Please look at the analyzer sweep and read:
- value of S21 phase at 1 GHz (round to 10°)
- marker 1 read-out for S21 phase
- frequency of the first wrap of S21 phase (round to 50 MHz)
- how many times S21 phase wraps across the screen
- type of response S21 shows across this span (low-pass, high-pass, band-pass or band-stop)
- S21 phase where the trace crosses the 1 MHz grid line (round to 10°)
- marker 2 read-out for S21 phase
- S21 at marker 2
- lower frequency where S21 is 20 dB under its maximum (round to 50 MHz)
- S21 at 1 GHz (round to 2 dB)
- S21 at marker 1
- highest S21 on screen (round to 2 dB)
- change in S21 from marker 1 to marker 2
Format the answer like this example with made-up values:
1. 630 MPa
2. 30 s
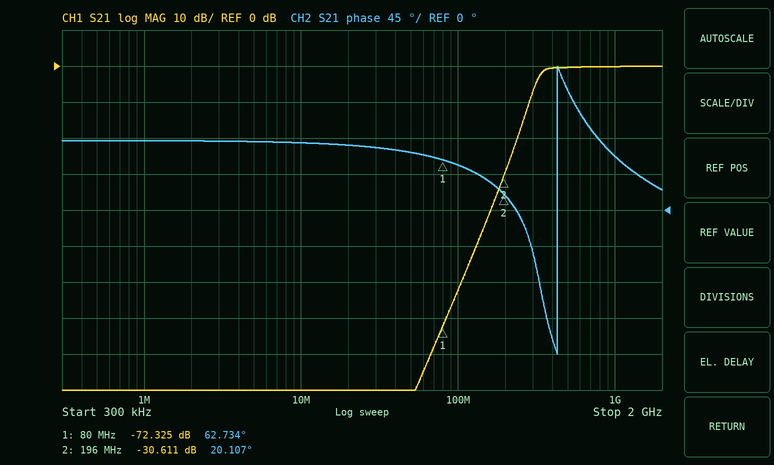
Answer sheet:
1. 70°
2. 62.734°
3. 450 MHz
4. 1
5. high-pass
6. 90°
7. 20.107°
8. -30.611 dB
9. 250 MHz
10. 0 dB
11. -72.325 dB
12. 0 dB
13. 41.714 dB
